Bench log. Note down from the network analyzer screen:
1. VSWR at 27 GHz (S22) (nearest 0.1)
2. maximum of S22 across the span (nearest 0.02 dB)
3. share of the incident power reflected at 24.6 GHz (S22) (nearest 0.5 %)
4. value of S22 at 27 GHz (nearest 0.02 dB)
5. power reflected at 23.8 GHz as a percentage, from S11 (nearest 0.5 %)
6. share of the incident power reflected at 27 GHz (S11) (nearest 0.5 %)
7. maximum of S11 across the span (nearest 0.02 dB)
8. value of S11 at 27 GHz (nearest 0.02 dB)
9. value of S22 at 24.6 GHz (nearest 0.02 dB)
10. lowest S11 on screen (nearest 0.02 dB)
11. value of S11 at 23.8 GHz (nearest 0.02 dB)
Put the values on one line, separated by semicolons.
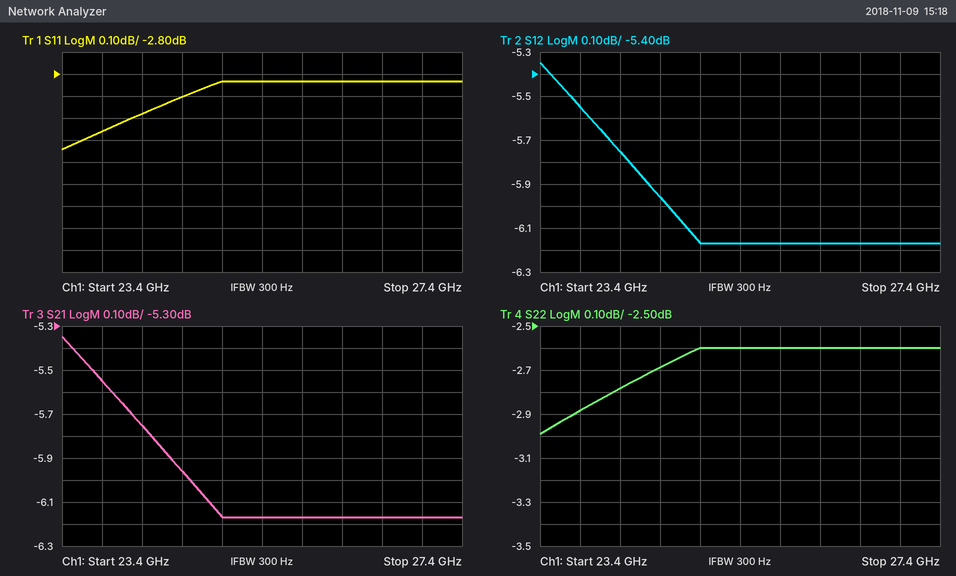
6.7; -2.60 dB; 54.0 %; -2.60 dB; 49.5 %; 52.0 %; -2.84 dB; -2.84 dB; -2.68 dB; -3.14 dB; -3.06 dB
